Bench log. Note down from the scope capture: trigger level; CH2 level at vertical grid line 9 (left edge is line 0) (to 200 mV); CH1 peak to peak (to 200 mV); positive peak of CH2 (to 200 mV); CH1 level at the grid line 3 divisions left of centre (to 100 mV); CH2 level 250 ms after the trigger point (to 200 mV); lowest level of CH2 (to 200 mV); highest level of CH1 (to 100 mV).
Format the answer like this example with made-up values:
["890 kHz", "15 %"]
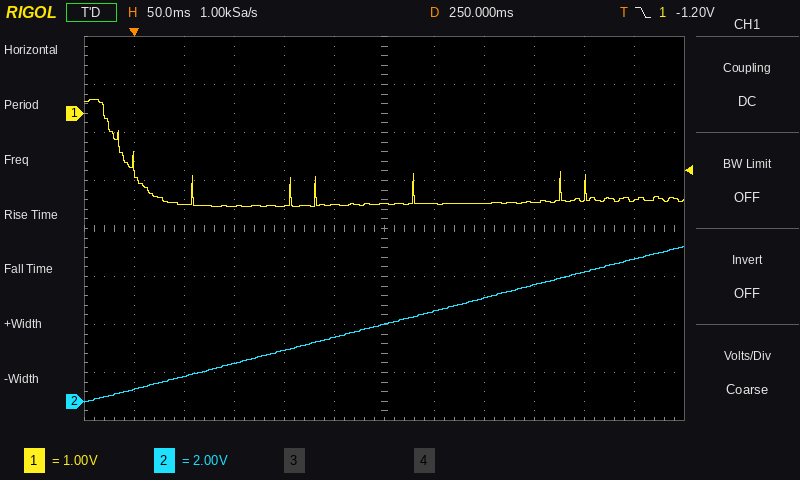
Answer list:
["-1.20 V", "4.8 V", "2.2 V", "6.4 V", "-1.9 V", "3.2 V", "0.0 V", "300 mV"]
